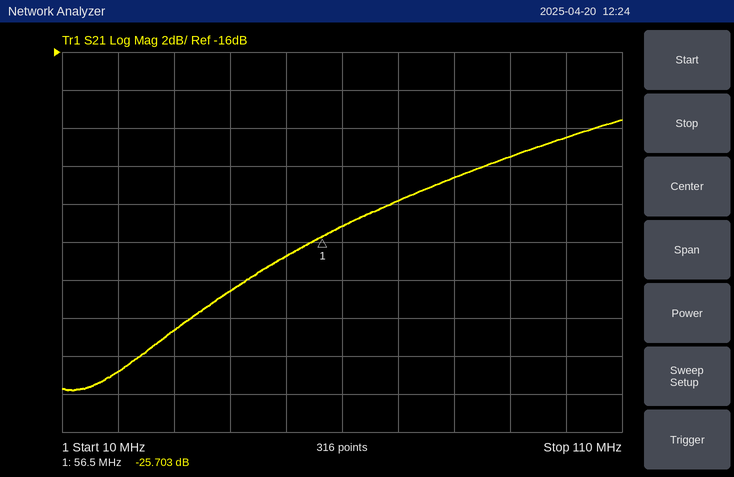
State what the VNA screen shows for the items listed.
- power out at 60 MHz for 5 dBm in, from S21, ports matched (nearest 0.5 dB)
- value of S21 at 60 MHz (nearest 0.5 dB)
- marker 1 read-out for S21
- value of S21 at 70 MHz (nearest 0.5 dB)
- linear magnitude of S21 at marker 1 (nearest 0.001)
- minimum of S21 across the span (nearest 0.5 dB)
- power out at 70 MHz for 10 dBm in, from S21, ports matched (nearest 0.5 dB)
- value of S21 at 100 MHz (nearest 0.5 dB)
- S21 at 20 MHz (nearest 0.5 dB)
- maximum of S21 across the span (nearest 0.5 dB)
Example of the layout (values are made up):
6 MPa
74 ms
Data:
-20.0 dBm
-25.0 dB
-25.703 dB
-24.0 dB
0.052
-34.0 dB
-14.0 dBm
-20.5 dB
-33.0 dB
-19.5 dB
